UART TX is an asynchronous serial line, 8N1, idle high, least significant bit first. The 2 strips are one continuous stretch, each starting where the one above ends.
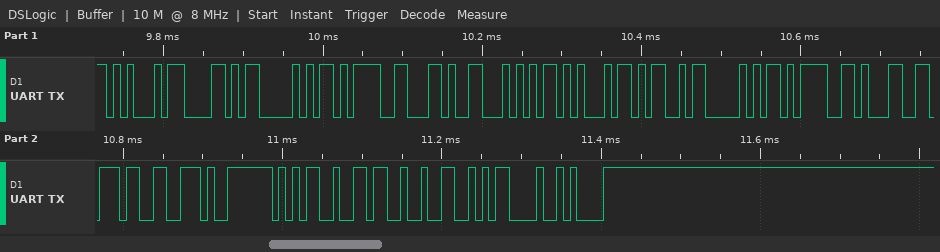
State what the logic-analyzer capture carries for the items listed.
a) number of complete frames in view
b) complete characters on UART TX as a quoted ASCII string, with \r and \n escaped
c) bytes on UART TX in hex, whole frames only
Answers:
18
"EXP=,TEMP=17.562\r\n"
45 58 50 3D 2C 54 45 4D 50 3D 31 37 2E 35 36 32 0D 0A
